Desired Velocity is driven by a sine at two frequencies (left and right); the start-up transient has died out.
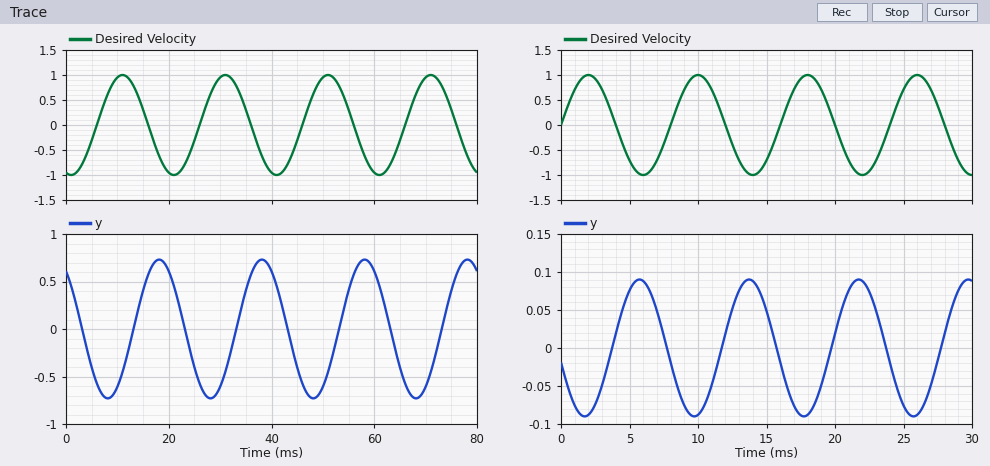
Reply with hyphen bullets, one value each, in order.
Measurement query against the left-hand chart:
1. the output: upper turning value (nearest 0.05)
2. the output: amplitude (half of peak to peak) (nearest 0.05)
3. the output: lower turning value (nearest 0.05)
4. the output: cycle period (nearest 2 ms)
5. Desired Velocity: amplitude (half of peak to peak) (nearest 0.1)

- 0.75
- 0.75
- -0.75
- 20 ms
- 1.0
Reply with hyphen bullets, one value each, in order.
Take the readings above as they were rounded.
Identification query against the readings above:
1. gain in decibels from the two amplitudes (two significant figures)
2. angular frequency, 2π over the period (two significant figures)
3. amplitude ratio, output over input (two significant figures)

- -2.5 dB
- 0.31 rad/ms
- 0.75
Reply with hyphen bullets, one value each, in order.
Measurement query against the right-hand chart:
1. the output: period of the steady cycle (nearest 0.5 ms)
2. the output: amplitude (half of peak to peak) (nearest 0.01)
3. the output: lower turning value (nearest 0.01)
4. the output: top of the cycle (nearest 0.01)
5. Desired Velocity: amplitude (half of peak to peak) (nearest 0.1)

- 8.0 ms
- 0.09
- -0.09
- 0.09
- 1.0
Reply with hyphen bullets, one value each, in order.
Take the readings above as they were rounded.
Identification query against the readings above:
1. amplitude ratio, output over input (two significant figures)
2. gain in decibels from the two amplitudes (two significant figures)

- 0.090
- -21 dB
